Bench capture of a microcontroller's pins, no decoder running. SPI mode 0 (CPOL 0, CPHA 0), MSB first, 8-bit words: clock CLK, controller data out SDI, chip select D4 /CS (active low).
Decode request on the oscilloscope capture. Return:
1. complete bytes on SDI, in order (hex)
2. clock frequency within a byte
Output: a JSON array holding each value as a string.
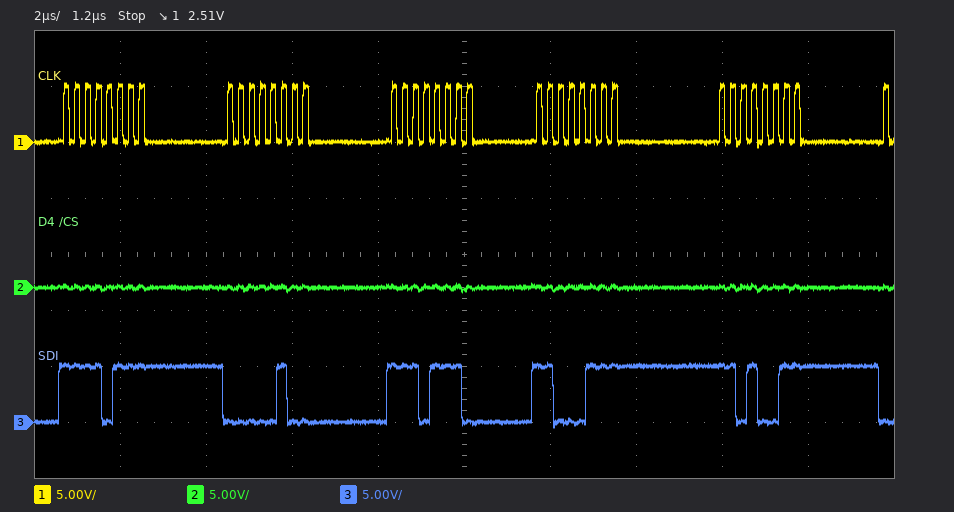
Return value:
["F7 04 EE C7 D3", "4 MHz"]
